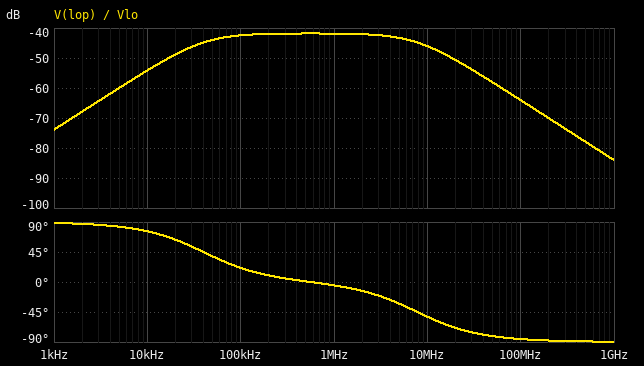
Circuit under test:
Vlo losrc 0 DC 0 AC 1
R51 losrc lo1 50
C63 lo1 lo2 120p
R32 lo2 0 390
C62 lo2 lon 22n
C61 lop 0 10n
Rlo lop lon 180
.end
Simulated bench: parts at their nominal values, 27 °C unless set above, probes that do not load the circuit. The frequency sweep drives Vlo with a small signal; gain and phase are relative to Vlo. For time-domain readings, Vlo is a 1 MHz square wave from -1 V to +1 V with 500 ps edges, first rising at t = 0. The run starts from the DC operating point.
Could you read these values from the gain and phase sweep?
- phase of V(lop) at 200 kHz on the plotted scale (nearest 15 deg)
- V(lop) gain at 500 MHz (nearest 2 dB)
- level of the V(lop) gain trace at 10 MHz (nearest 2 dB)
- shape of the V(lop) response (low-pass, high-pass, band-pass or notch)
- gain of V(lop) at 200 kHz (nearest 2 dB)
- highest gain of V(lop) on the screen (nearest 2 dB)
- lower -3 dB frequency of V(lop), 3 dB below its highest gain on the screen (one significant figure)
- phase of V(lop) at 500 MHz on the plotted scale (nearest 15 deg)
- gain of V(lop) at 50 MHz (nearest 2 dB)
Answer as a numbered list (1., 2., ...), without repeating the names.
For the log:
1. 15 deg
2. -78 dB
3. -46 dB
4. band-pass
5. -42 dB
6. -42 dB
7. 40 kHz
8. -90 deg
9. -58 dB
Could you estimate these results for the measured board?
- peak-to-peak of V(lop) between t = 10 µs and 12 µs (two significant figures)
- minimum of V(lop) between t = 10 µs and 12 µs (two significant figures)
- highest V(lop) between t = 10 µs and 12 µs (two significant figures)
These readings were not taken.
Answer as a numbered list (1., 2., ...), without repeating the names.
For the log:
1. 17 mV
2. -8.0 mV
3. 9.0 mV
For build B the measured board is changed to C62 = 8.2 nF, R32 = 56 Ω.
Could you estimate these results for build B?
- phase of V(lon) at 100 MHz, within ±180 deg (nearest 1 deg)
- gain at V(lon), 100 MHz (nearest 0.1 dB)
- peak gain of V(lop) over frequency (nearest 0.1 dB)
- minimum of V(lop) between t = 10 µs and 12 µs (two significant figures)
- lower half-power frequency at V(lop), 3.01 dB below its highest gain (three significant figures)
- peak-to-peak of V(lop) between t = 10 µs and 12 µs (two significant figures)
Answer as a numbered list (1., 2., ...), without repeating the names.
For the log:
1. 8 deg
2. -6.8 dB
3. -51.0 dB
4. -3.3 mV
5. 146 kHz
6. 6.6 mV
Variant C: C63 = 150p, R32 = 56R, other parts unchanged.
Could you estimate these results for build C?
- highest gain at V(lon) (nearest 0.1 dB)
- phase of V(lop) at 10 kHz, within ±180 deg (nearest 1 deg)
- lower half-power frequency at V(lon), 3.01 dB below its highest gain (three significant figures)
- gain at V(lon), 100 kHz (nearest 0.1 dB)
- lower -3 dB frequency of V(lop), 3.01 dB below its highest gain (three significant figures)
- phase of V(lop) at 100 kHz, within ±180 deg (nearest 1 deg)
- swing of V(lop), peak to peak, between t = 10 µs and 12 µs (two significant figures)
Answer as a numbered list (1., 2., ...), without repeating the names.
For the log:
1. -6.7 dB
2. 84 deg
3. 11.5 MHz
4. -48.3 dB
5. 96.3 kHz
6. 44 deg
7. 7.8 mV
